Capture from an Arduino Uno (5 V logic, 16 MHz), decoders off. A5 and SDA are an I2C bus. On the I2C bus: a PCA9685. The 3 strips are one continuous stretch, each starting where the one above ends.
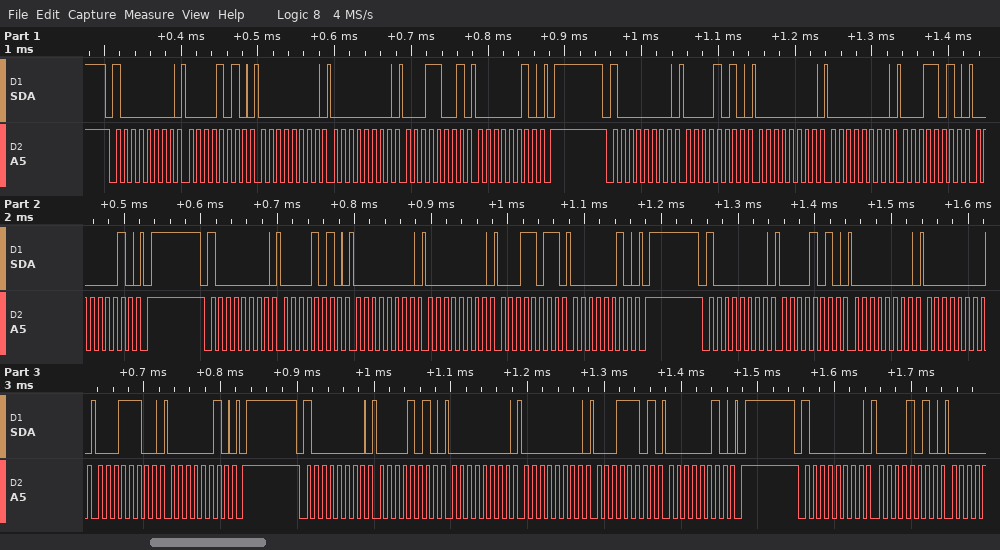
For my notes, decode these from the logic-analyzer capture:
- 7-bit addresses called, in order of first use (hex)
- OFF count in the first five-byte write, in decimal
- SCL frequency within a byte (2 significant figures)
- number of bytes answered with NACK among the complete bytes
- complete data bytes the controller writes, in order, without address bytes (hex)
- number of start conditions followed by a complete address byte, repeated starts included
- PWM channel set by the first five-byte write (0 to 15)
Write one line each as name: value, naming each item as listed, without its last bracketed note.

7-bit addresses called, in order of first use: 0x40
OFF count in the first five-byte write, in decimal: 537
SCL frequency within a byte: 100 kHz
number of bytes answered with NACK among the complete bytes: 0
complete data bytes the controller writes, in order, without address bytes: 0A 00 00 19 02 0A 00 00 1A 02 0A 00 00 1B 02 0A 00 00 1C 02 0A 00 00 1D 02 0A
number of start conditions followed by a complete address byte, repeated starts included: 6
PWM channel set by the first five-byte write: 1
